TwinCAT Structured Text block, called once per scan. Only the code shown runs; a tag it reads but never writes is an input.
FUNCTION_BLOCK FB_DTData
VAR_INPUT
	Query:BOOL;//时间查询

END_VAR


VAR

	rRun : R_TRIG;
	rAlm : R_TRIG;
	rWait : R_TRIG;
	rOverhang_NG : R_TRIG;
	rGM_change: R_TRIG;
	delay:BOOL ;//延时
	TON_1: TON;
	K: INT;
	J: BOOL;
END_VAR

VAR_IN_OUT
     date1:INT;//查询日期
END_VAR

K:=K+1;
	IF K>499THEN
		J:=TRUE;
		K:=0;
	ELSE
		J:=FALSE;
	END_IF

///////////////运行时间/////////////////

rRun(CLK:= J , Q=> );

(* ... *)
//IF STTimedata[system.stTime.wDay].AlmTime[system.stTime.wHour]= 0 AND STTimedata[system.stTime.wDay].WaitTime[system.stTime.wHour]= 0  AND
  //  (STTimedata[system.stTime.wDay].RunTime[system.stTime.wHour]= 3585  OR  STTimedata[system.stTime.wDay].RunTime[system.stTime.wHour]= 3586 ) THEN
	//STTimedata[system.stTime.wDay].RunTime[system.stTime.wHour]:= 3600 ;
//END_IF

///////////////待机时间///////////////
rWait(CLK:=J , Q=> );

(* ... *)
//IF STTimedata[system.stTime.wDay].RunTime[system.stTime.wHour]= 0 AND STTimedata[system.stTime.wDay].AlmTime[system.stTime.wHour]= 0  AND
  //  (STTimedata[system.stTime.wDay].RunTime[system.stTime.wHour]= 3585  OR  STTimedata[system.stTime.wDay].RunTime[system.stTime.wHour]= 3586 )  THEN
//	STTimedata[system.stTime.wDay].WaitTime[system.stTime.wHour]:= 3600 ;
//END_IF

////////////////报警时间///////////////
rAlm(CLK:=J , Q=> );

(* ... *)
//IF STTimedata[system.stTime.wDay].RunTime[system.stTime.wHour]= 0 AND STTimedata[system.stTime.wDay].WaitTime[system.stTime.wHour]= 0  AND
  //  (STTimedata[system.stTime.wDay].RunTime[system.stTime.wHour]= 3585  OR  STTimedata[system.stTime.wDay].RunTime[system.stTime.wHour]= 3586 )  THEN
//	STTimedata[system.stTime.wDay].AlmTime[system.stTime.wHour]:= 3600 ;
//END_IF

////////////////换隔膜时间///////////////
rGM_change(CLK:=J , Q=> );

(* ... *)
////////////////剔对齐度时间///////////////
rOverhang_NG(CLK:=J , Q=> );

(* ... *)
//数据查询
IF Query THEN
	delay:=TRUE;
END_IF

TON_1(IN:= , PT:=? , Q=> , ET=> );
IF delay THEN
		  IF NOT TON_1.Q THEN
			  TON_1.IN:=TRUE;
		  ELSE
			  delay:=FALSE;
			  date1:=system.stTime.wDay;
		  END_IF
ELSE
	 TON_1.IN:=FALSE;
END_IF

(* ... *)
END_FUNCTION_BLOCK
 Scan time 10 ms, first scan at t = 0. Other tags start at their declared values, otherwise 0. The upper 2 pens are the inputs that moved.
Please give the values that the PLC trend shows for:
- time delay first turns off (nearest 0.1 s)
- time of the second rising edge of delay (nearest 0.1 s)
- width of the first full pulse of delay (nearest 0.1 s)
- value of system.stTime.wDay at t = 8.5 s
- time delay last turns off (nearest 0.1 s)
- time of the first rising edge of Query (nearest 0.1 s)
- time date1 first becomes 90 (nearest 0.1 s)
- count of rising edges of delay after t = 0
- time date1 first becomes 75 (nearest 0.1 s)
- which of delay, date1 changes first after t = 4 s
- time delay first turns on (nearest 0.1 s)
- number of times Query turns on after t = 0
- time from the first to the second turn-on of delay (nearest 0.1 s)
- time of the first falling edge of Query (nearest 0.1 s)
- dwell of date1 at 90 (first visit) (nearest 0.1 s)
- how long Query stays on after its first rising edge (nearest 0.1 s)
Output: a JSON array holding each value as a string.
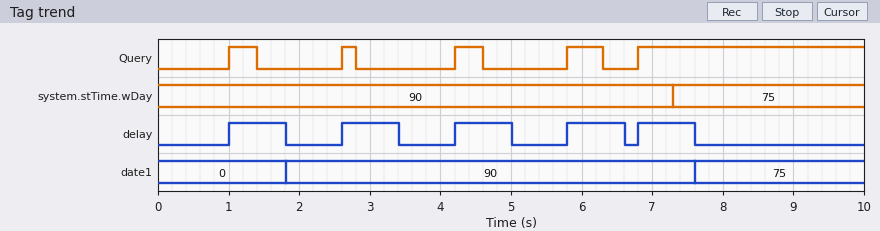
["1.8 s", "2.6 s", "0.8 s", "75", "7.6 s", "1.0 s", "1.8 s", "5", "7.6 s", "delay", "1.0 s", "5", "1.6 s", "1.4 s", "5.8 s", "0.4 s"]
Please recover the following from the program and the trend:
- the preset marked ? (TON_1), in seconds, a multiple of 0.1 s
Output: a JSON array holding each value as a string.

["0.8 s"]
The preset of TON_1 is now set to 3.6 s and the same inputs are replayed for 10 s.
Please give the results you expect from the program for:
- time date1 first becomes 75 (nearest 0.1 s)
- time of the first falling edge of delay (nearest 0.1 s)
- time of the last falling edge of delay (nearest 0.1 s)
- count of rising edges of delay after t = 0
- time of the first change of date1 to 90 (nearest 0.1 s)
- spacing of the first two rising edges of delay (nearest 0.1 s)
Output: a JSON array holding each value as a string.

["9.4 s", "4.6 s", "9.4 s", "2", "4.6 s", "4.8 s"]
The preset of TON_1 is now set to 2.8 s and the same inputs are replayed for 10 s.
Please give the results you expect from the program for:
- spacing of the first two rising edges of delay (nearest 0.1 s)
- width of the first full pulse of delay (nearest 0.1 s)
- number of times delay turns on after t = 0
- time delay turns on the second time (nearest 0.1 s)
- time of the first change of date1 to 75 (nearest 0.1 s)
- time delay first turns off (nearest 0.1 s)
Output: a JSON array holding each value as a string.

["3.2 s", "2.8 s", "2", "4.2 s", "7.3 s", "3.8 s"]
